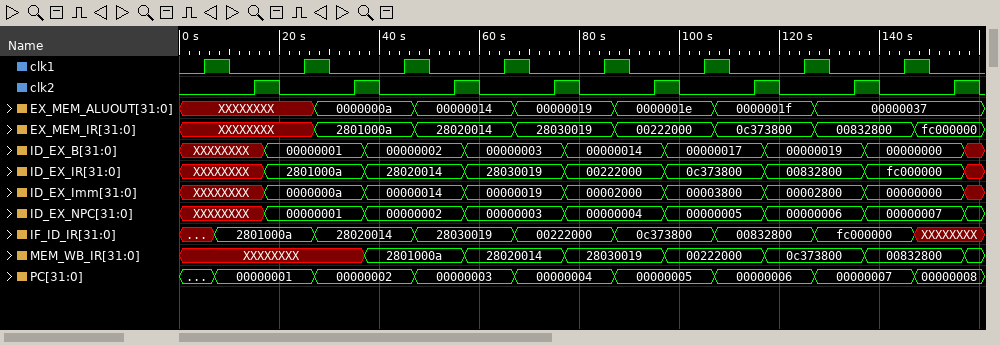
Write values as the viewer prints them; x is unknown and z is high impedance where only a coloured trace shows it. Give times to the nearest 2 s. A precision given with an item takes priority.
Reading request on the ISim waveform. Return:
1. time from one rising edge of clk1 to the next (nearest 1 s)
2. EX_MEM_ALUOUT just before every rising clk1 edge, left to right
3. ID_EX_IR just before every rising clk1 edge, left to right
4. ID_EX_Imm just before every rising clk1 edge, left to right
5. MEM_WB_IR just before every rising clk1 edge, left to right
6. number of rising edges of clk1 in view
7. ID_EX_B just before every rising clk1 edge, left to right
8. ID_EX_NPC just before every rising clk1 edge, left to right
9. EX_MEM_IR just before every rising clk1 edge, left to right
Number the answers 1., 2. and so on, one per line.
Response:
1. 20 s
2. XXXXXXXX, XXXXXXXX, 0000000a, 00000014, 00000019, 0000001e, 0000001f, 00000037
3. XXXXXXXX, 2801000a, 28020014, 28030019, 00222000, 0c373800, 00832800, fc000000
4. XXXXXXXX, 0000000a, 00000014, 00000019, 00002000, 00003800, 00002800, 00000000
5. XXXXXXXX, XXXXXXXX, 2801000a, 28020014, 28030019, 00222000, 0c373800, 00832800
6. 8
7. XXXXXXXX, 00000001, 00000002, 00000003, 00000014, 00000017, 00000019, 00000000
8. XXXXXXXX, 00000001, 00000002, 00000003, 00000004, 00000005, 00000006, 00000007
9. XXXXXXXX, XXXXXXXX, 2801000a, 28020014, 28030019, 00222000, 0c373800, 00832800
